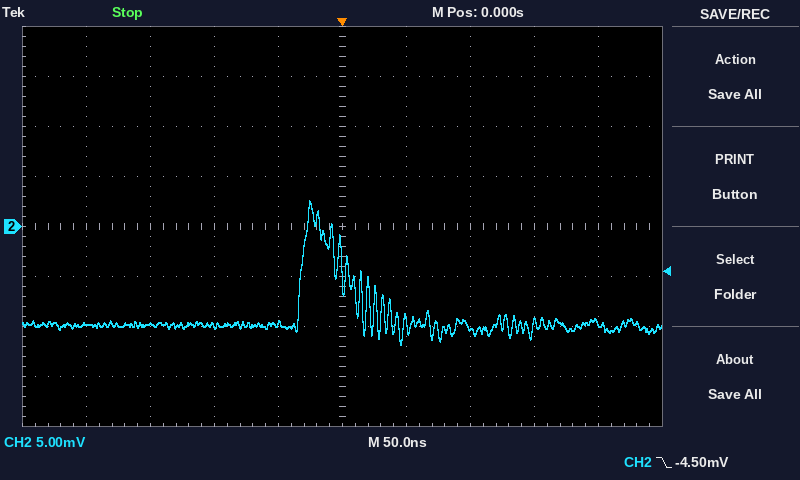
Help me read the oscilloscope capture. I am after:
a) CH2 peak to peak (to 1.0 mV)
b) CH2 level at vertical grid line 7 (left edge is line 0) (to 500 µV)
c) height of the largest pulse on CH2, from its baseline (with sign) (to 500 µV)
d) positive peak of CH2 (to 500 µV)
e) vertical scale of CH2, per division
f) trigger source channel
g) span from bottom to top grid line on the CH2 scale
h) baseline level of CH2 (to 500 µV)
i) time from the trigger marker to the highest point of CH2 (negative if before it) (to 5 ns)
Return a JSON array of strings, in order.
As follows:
["14.0 mV", "-10.0 mV", "+12.5 mV", "2.5 mV", "5 mV", "CH2", "40 mV", "-10.0 mV", "-25 ns"]
